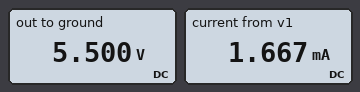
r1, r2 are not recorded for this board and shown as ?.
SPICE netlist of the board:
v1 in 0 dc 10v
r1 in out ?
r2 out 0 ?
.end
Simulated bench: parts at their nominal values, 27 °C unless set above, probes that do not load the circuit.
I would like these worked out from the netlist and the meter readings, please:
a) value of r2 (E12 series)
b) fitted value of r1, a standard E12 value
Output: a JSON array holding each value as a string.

["3.3 kΩ", "2.7 kΩ"]
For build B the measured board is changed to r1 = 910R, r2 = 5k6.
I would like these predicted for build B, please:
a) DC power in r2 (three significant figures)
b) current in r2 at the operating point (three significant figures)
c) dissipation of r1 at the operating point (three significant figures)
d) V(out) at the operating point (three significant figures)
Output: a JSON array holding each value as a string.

["13.2 mW", "1.54 mA", "2.15 mW", "8.60 V"]
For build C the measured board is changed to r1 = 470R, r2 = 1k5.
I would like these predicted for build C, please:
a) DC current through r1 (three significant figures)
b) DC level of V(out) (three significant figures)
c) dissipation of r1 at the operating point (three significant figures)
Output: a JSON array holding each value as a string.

["5.08 mA", "7.61 V", "12.1 mW"]
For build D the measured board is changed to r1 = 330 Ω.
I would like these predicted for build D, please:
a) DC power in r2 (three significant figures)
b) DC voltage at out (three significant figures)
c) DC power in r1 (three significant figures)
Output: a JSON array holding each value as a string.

["25.0 mW", "9.09 V", "2.50 mW"]
